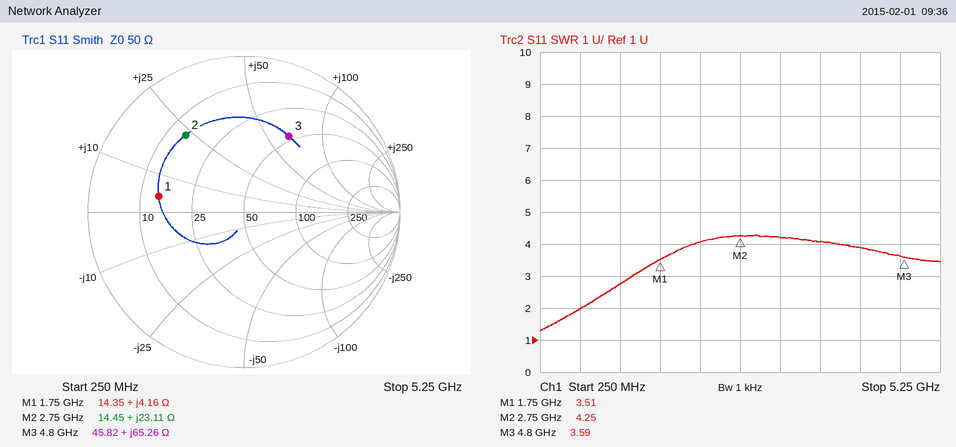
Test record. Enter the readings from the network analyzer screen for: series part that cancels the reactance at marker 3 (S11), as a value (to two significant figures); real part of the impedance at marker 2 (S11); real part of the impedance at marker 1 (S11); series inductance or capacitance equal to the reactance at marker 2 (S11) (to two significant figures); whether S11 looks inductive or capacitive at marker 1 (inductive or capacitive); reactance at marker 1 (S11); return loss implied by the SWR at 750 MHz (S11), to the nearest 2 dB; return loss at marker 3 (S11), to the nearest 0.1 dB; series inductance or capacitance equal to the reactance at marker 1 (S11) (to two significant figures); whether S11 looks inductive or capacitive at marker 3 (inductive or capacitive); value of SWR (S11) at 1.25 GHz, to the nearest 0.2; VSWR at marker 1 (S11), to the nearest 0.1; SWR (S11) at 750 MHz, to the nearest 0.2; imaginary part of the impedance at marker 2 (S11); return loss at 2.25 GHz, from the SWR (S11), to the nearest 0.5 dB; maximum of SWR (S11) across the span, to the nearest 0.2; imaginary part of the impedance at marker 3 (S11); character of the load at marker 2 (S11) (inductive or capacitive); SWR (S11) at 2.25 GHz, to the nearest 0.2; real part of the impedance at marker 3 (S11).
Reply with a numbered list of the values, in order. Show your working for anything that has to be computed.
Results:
1. C = 1/(2π × 4.8 GHz × 65.26 Ω) ≈ 508 fF, so 510 fF to two significant figures
2. 14.45 Ω
3. 14.35 Ω
4. L = 23.11 Ω/(2π × 2.75 GHz) ≈ 1.3 nH
5. inductive
6. +4.16 Ω
7. −20 log10((2 − 1)/(2 + 1)) ≈ 10 dB
8. 5.0 dB
9. L = 4.16 Ω/(2π × 1.75 GHz) ≈ 378 pH, so 380 pH to two significant figures
10. inductive
11. 2.8
12. 3.5
13. 2.0
14. +23.11 Ω
15. −20 log10((4 − 1)/(4 + 1)) ≈ 4.44 dB, so 4.5 dB to the nearest 0.5 dB
16. 4.2
17. +65.26 Ω
18. inductive
19. 4.0
20. 45.82 Ω
